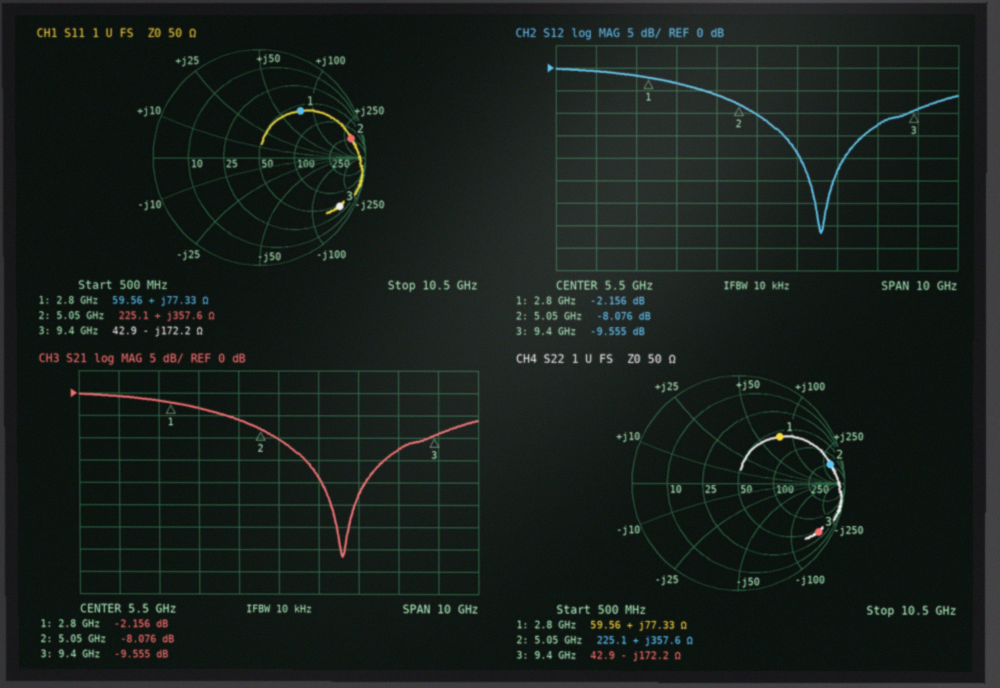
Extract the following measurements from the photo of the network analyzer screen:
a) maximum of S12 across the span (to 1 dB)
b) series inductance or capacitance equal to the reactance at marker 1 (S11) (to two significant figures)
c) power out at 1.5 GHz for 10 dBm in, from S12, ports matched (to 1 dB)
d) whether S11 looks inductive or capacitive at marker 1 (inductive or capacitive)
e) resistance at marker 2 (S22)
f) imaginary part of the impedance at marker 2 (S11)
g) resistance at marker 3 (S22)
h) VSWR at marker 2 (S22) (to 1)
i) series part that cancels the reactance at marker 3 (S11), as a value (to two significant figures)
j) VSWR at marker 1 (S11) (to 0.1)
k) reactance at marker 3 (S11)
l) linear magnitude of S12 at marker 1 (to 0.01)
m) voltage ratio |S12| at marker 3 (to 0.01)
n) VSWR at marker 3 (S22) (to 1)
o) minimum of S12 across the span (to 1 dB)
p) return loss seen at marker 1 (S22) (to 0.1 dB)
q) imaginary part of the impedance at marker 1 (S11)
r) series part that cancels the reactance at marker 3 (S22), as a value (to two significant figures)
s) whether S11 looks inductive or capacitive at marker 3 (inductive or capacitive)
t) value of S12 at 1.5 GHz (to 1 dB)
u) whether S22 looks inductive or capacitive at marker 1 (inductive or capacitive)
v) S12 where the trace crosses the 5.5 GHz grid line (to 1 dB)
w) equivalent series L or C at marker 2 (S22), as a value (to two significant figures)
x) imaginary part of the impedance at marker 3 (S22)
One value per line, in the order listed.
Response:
0 dB
4.4 nH
9 dBm
inductive
225.1 Ω
+357.6 Ω
42.9 Ω
16
2.9 nH
3.8
-172.2 Ω
0.78
0.33
16
-37 dB
4.7 dB
+77.33 Ω
2.9 nH
capacitive
-1 dB
inductive
-10 dB
11 nH
-172.2 Ω
